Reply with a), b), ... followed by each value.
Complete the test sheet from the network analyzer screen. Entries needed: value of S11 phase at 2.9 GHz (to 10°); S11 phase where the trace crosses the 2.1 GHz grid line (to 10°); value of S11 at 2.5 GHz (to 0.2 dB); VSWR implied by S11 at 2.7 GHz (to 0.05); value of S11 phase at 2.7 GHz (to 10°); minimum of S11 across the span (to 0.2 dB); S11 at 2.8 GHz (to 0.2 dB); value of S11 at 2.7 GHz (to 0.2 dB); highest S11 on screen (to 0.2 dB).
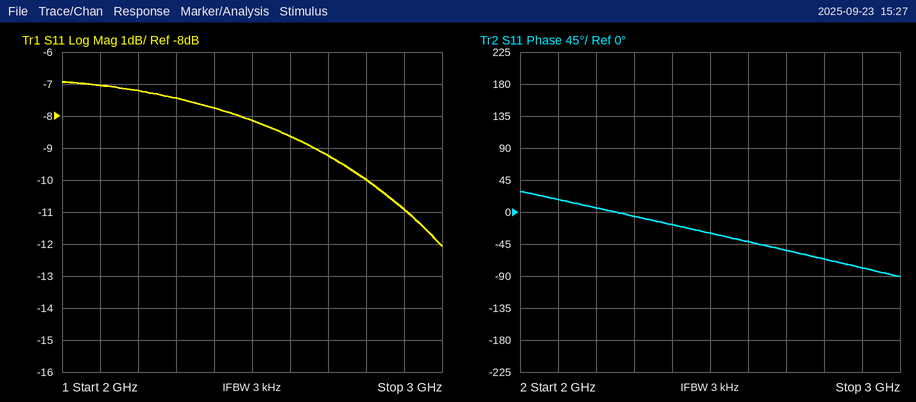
a) -80°
b) 20°
c) -8.2 dB
d) 2.05
e) -50°
f) -12.0 dB
g) -10.0 dB
h) -9.2 dB
i) -7.0 dB
